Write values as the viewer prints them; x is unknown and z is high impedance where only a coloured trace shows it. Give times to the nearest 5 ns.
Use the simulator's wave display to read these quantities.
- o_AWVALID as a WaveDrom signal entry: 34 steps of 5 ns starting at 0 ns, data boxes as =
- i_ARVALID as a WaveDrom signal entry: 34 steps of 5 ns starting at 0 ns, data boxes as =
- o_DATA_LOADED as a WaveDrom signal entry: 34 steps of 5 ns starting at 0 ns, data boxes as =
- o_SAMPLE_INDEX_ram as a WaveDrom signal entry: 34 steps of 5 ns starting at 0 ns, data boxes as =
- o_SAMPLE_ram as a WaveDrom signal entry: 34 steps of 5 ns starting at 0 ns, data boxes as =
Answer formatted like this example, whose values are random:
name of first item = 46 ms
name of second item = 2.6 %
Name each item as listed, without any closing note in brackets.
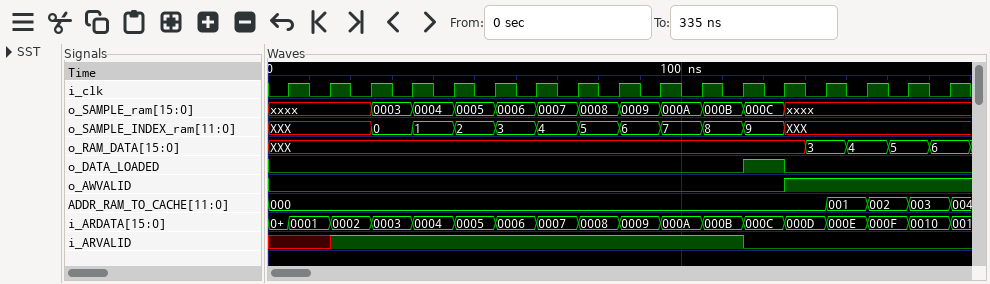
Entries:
o_AWVALID as a WaveDrom signal entry: 34 steps of 5 ns starting at 0 ns, data boxes as = = {name: 'o_AWVALID', wave: '0........................1........'}
i_ARVALID as a WaveDrom signal entry: 34 steps of 5 ns starting at 0 ns, data boxes as = = {name: 'i_ARVALID', wave: 'x..1...................0..........'}
o_DATA_LOADED as a WaveDrom signal entry: 34 steps of 5 ns starting at 0 ns, data boxes as = = {name: 'o_DATA_LOADED', wave: '0......................1.0........'}
o_SAMPLE_INDEX_ram as a WaveDrom signal entry: 34 steps of 5 ns starting at 0 ns, data boxes as = = {name: 'o_SAMPLE_INDEX_ram', wave: 'x....=.=.=.=.=.=.=.=.=.=.x........', data: '0 1 2 3 4 5 6 7 8 9'}
o_SAMPLE_ram as a WaveDrom signal entry: 34 steps of 5 ns starting at 0 ns, data boxes as = = {name: 'o_SAMPLE_ram', wave: 'x....=.=.=.=.=.=.=.=.=.=.x........', data: '0003 0004 0005 0006 0007 0008 0009 000A 000B 000C'}
